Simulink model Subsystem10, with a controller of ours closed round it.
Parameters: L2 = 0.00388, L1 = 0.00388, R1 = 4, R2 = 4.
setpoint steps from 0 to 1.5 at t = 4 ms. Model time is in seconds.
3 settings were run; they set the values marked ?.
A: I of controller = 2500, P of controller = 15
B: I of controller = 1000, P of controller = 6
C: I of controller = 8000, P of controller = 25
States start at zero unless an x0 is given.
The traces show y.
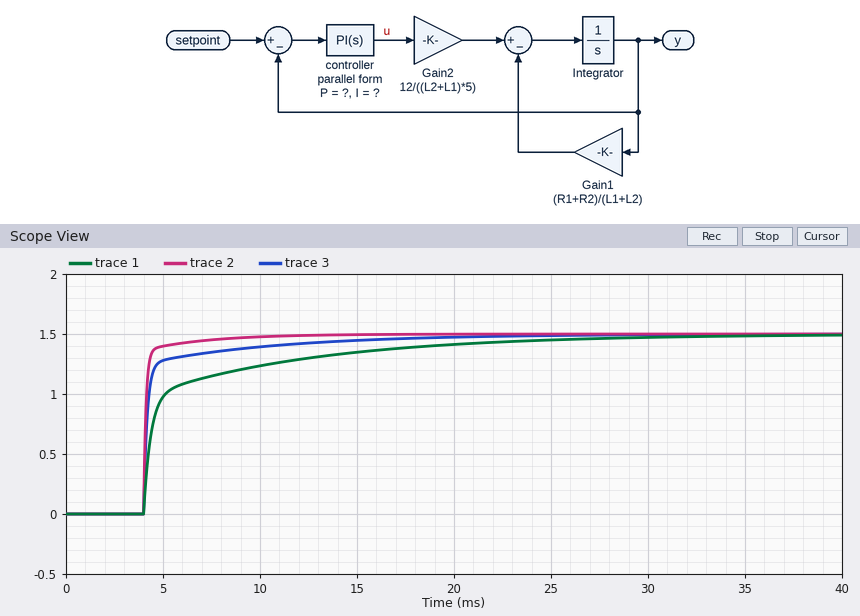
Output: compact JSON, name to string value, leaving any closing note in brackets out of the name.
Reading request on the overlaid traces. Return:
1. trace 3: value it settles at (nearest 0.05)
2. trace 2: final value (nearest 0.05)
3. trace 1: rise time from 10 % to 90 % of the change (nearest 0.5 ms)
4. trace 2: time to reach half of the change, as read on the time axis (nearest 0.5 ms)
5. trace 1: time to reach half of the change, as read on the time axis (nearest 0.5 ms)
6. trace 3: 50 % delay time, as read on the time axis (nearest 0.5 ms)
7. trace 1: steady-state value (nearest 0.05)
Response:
{"trace 3: value it settles at": "1.50", "trace 2: final value": "1.50", "trace 1: rise time from 10 % to 90 % of the change": "11.0 ms", "trace 2: time to reach half of the change, as read on the time axis": "4.0 ms", "trace 1: time to reach half of the change, as read on the time axis": "4.5 ms", "trace 3: 50 % delay time, as read on the time axis": "4.0 ms", "trace 1: steady-state value": "1.50"}
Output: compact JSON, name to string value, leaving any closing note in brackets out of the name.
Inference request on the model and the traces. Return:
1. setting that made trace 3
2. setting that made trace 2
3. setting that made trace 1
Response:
{"setting that made trace 3": "A", "setting that made trace 2": "C", "setting that made trace 1": "B"}
